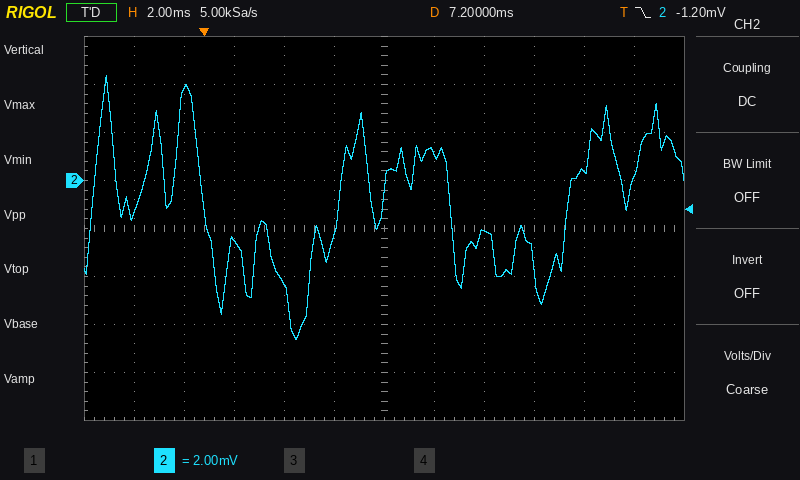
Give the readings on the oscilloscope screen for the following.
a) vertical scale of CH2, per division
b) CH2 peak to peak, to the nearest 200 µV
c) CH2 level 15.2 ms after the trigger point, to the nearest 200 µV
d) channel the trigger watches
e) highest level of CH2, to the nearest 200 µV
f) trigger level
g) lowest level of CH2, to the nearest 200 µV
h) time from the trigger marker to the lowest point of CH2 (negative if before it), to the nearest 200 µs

2 mV
11.0 mV
400 µV
CH2
4.4 mV
-1.20 mV
-6.6 mV
+3.6 ms
